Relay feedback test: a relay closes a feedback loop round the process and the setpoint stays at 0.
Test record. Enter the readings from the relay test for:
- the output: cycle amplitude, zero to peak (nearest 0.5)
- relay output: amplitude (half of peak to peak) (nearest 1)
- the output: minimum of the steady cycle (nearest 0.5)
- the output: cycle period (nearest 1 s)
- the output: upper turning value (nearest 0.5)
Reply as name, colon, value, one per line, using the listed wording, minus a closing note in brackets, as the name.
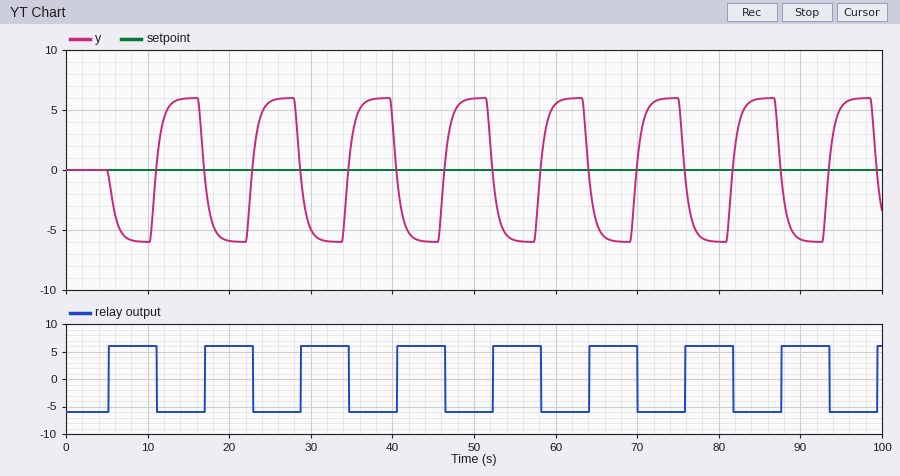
the output: cycle amplitude, zero to peak: 6.0
relay output: amplitude (half of peak to peak): 6
the output: minimum of the steady cycle: -6.0
the output: cycle period: 12 s
the output: upper turning value: 6.0
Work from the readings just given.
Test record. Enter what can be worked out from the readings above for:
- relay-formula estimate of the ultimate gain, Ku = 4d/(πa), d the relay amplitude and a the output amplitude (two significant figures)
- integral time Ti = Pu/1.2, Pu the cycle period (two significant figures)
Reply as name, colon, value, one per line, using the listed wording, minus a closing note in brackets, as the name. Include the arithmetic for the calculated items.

relay-formula estimate of the ultimate gain, Ku = 4d/(πa), d the relay amplitude and a the output amplitude: 4 × 6 / (π × 6) = 1.3
integral time Ti = Pu/1.2, Pu the cycle period: 12 / 1.2 = 10 s
